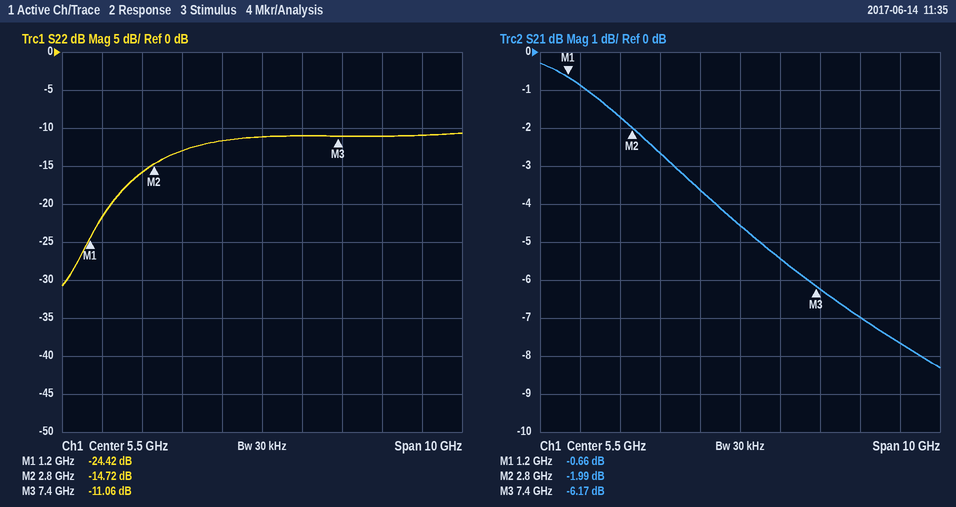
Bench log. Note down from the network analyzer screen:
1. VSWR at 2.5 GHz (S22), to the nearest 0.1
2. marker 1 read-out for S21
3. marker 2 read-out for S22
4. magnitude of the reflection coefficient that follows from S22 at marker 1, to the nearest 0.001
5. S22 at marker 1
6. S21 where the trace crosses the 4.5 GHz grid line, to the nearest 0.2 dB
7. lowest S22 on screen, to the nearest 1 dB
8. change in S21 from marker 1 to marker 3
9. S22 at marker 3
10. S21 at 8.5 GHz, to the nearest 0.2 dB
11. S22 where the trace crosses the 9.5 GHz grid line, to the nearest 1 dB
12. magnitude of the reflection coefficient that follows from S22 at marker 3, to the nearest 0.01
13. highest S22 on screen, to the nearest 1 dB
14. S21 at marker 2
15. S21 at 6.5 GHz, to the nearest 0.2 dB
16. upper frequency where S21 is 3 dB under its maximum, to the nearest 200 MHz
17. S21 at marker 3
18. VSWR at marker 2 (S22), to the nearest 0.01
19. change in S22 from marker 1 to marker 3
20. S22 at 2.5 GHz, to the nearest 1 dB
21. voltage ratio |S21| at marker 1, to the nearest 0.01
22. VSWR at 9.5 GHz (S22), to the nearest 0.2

1.4
-0.66 dB
-14.72 dB
0.060
-24.42 dB
-3.6 dB
-31 dB
-5.51 dB
-11.06 dB
-7.0 dB
-11 dB
0.28
-11 dB
-1.99 dB
-5.4 dB
4.2 GHz
-6.17 dB
1.45
13.36 dB
-16 dB
0.93
1.8
